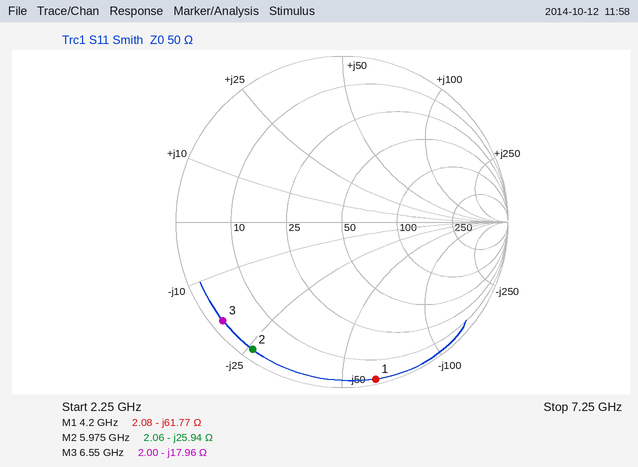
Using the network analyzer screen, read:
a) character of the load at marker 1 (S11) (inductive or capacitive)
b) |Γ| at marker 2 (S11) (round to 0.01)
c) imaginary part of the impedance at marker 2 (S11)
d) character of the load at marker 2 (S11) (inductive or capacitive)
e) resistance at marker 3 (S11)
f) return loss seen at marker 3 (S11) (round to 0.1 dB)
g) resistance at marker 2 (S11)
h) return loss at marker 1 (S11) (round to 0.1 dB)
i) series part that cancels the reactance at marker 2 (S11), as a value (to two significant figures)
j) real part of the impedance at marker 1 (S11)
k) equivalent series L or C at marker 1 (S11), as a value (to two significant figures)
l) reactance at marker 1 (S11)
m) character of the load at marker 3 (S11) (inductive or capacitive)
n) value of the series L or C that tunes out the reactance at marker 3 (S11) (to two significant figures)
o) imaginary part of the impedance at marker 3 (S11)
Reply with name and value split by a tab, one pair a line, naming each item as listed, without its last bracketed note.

character of the load at marker 1 (S11)	capacitive
|Γ| at marker 2 (S11)	0.94
imaginary part of the impedance at marker 2	-25.94 Ω
character of the load at marker 2 (S11)	capacitive
resistance at marker 3	2.00 Ω
return loss seen at marker 3 (S11)	0.6 dB
resistance at marker 2	2.06 Ω
return loss at marker 1 (S11)	0.3 dB
series part that cancels the reactance at marker 2 (S11), as a value	690 pH
real part of the impedance at marker 1	2.08 Ω
equivalent series L or C at marker 1 (S11), as a value	610 fF
reactance at marker 1	-61.77 Ω
character of the load at marker 3 (S11)	capacitive
value of the series L or C that tunes out the reactance at marker 3 (S11)	440 pH
imaginary part of the impedance at marker 3	-17.96 Ω
